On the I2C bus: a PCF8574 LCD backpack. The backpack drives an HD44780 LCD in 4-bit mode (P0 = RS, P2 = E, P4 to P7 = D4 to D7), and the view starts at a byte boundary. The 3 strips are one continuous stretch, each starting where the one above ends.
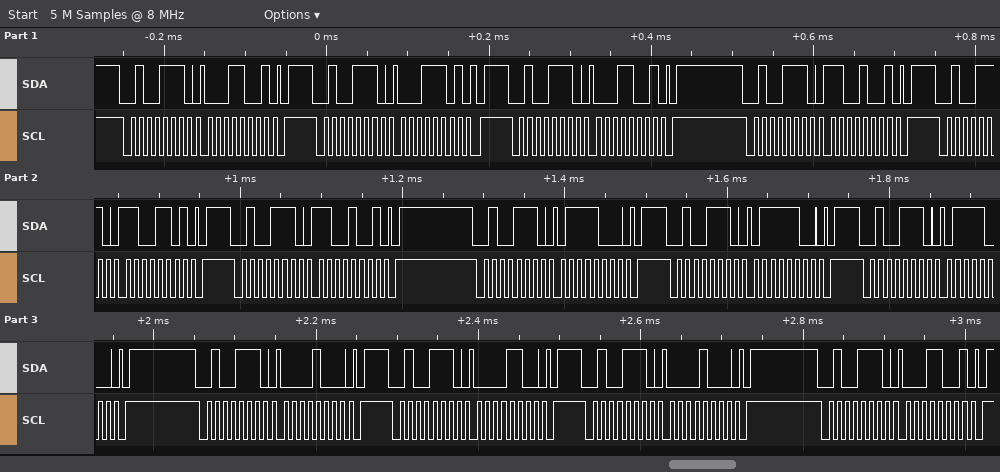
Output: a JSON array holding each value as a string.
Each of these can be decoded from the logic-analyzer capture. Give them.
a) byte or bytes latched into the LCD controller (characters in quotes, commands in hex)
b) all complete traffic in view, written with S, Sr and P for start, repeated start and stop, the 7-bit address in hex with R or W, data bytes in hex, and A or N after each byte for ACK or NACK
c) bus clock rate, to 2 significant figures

["data 0x1C 0x70", "S 27W A 19 A P S 27W A 1D A P S 27W A 19 A P S 27W A C9 A P S 27W A CD A P S 27W A C9 A P S 27W A 78 A P S 27W A 7C A P S 27W A 78 A P S 27W A 08 A P S 27W A 0C A P S 27W A 08 A P S 27W A 19 A P", "100 kHz"]
